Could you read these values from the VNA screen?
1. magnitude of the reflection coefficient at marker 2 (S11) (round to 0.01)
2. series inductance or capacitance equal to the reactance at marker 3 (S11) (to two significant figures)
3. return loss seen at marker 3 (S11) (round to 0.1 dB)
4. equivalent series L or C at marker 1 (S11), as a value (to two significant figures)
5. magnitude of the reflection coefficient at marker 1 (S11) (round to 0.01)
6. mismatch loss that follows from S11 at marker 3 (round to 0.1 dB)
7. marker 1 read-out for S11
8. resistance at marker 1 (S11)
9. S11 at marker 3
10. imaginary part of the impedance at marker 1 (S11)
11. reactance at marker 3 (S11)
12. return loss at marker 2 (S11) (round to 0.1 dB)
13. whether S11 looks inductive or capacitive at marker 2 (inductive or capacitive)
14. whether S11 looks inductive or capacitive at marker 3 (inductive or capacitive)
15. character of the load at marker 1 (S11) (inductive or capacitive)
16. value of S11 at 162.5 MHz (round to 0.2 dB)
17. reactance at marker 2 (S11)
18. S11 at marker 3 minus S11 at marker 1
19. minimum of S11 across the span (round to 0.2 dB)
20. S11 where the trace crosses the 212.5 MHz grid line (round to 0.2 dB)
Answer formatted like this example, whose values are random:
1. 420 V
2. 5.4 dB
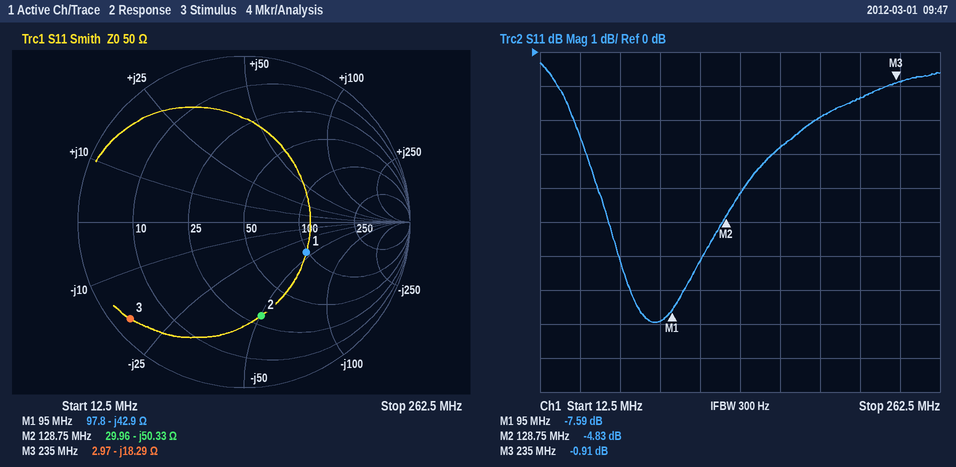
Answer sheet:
1. 0.57
2. 37 pF
3. 0.9 dB
4. 39 pF
5. 0.42
6. 7.2 dB
7. -7.59 dB
8. 97.8 Ω
9. -0.91 dB
10. -42.9 Ω
11. -18.29 Ω
12. 4.8 dB
13. capacitive
14. capacitive
15. capacitive
16. -2.8 dB
17. -50.33 Ω
18. 6.68 dB
19. -8.0 dB
20. -1.4 dB
